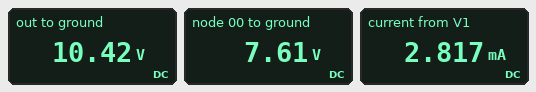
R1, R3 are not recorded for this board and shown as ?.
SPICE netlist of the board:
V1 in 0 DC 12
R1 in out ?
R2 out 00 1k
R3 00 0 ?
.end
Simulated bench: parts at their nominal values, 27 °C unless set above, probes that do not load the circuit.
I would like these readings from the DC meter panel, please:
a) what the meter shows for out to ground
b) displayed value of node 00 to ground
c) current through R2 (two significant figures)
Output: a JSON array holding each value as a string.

["10.42 V", "7.61 V", "2.8 mA"]
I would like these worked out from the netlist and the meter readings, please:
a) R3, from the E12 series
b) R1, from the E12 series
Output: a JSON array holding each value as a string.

["2.7 kΩ", "560 Ω"]
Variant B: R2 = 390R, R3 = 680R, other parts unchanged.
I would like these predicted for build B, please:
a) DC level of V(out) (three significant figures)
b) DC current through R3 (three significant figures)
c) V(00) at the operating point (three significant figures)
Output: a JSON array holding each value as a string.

["7.88 V", "7.36 mA", "5.01 V"]
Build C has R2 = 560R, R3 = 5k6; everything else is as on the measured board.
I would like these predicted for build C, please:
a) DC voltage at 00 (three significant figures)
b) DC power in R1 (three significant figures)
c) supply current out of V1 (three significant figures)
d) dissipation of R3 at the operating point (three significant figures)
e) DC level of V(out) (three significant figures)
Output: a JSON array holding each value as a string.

["10.0 V", "1.79 mW", "1.79 mA", "17.9 mW", "11.0 V"]
